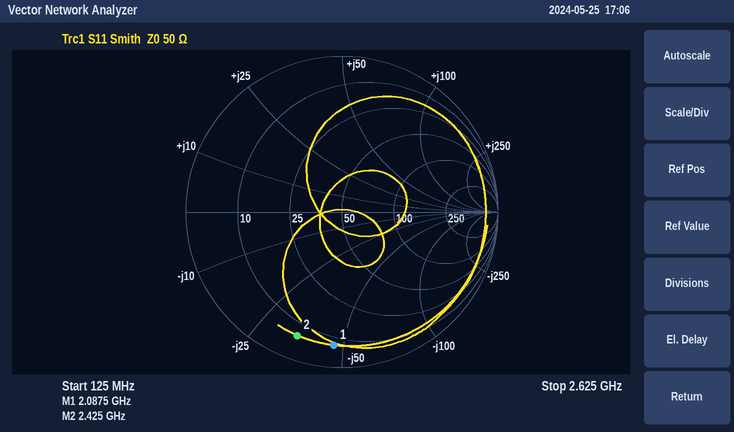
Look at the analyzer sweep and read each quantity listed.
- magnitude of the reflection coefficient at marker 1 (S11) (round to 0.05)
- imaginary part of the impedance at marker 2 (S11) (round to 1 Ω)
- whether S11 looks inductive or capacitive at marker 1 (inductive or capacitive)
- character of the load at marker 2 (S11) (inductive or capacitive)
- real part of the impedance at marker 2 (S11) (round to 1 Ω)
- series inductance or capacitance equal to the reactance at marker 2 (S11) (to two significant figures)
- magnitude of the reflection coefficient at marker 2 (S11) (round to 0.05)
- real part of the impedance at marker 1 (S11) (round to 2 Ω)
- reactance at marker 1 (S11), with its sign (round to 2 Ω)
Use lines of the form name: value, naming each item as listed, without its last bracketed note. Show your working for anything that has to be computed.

magnitude of the reflection coefficient at marker 1 (S11): 0.85
imaginary part of the impedance at marker 2 (S11): -35 Ω
whether S11 looks inductive or capacitive at marker 1: capacitive
character of the load at marker 2 (S11): capacitive
real part of the impedance at marker 2 (S11): 6 Ω
series inductance or capacitance equal to the reactance at marker 2 (S11): C = 1/(2π × 2.425 GHz × 35 Ω) ≈ 1.9 pF
magnitude of the reflection coefficient at marker 2 (S11): 0.85
real part of the impedance at marker 1 (S11): 8 Ω
reactance at marker 1 (S11), with its sign: -46 Ω
